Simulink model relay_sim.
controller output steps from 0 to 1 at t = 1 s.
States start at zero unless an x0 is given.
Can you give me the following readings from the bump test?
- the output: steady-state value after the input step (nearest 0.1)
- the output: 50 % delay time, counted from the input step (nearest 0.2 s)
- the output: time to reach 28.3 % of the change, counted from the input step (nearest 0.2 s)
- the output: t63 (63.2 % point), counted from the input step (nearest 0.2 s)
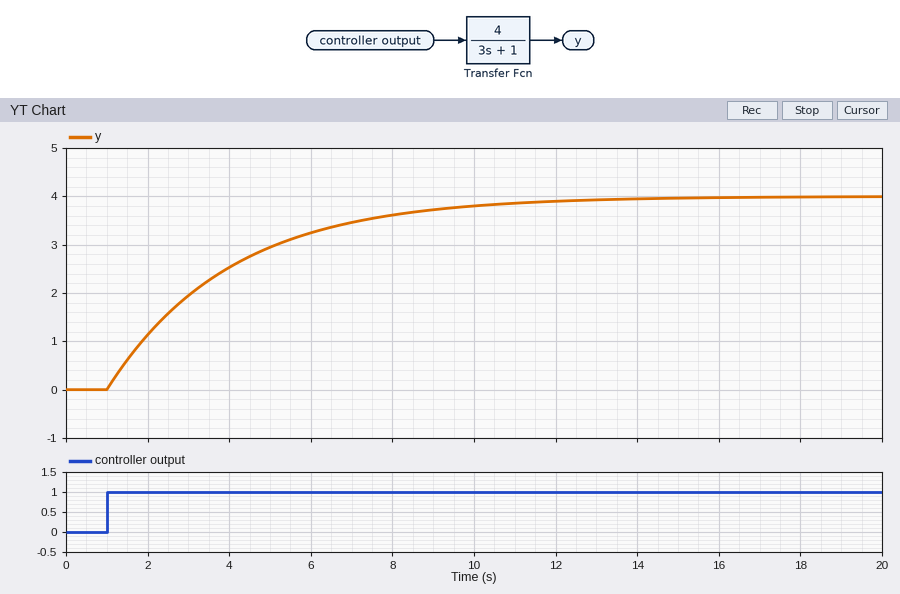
4.0
2.0 s
1.0 s
3.0 s
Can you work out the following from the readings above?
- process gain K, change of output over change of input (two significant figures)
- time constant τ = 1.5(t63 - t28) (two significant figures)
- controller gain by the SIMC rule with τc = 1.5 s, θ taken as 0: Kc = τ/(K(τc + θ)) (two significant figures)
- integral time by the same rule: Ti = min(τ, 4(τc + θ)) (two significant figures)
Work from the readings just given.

4.0
3.0 s
0.50
3.0 s
